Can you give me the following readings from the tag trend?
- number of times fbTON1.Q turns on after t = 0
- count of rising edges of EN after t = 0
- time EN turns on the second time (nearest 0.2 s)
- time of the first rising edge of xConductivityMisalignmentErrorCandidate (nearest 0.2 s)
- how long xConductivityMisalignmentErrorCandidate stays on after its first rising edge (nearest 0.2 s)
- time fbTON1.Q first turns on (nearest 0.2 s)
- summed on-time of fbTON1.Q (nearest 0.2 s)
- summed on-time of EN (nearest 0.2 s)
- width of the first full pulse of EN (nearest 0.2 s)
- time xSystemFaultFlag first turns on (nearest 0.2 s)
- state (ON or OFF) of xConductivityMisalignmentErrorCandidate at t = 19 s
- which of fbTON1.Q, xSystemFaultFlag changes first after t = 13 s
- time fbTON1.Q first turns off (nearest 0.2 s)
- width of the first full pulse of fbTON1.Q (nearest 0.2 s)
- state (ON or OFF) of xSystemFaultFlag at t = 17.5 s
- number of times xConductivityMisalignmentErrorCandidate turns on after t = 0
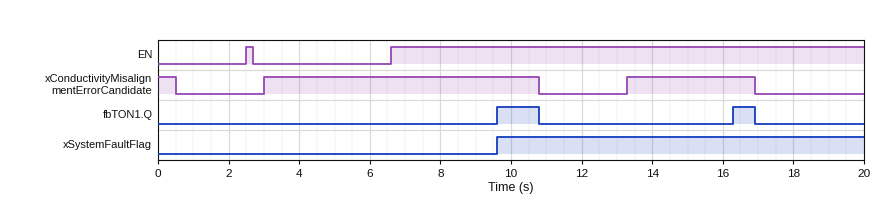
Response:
2
2
6.6 s
3.0 s
7.8 s
9.6 s
1.8 s
13.6 s
0.2 s
9.6 s
OFF
fbTON1.Q
10.8 s
1.2 s
ON
2
